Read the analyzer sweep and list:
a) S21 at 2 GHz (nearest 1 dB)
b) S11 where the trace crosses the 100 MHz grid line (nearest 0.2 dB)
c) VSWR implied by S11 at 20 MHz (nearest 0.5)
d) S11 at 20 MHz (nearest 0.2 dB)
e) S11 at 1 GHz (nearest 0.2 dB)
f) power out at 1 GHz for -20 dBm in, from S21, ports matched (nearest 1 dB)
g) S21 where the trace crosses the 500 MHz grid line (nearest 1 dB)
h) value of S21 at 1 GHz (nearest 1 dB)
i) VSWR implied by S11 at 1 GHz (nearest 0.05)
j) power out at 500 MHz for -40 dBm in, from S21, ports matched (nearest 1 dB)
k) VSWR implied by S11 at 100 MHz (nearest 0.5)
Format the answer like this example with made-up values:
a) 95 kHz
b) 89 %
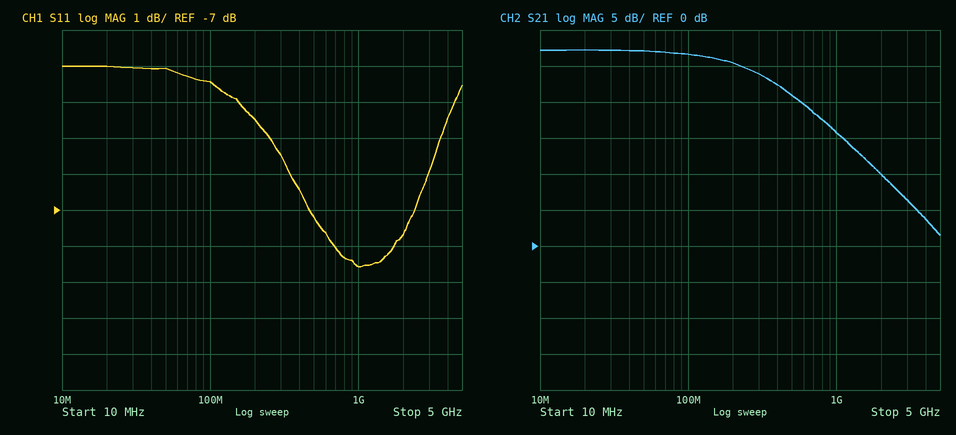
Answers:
a) 10 dB
b) -3.4 dB
c) 6.0
d) -3.0 dB
e) -8.6 dB
f) -4 dBm
g) 21 dB
h) 16 dB
i) 2.20
j) -19 dBm
k) 5.0
